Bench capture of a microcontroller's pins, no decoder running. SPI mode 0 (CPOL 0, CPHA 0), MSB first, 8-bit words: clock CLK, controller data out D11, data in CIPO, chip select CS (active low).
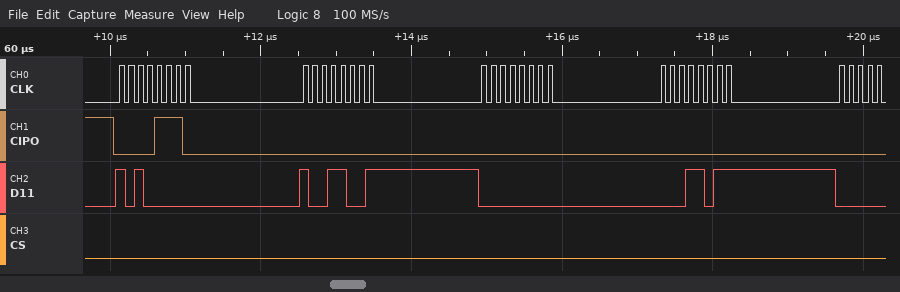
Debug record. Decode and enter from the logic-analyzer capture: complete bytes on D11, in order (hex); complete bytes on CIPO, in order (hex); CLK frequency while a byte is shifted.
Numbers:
0xA0 0x99 0x00 0x1B
0x0E 0x00 0x00 0x00
8 MHz
